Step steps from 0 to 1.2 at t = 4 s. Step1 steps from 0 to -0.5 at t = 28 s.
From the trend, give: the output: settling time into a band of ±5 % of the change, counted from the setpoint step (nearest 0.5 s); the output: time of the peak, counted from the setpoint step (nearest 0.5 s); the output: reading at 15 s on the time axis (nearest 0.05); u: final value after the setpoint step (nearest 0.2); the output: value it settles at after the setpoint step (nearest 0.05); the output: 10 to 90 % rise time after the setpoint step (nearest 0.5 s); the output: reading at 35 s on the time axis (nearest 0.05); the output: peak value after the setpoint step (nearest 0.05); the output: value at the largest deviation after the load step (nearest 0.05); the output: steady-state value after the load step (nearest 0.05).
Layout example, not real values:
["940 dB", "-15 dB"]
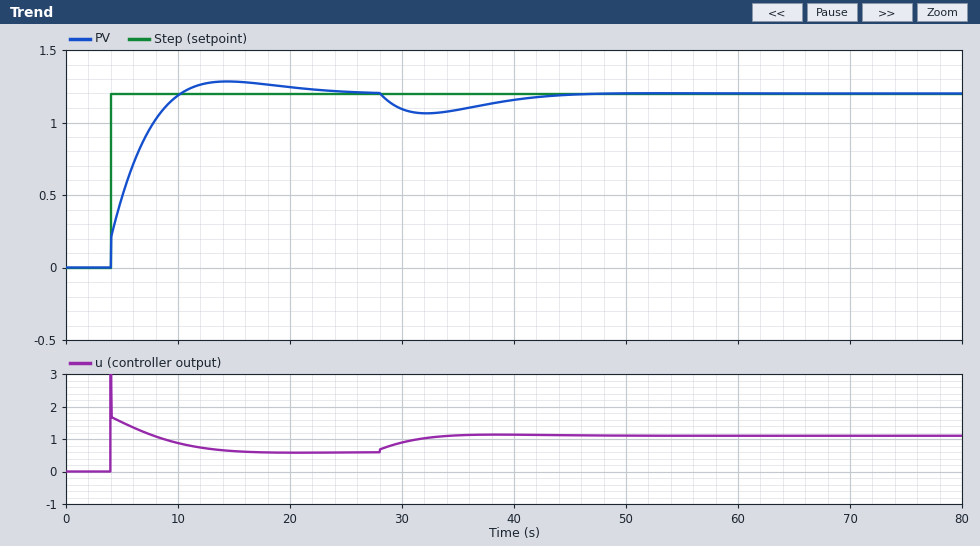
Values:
["14.0 s", "10.5 s", "1.30", "0.6", "1.20", "4.5 s", "1.10", "1.30", "1.05", "1.20"]
